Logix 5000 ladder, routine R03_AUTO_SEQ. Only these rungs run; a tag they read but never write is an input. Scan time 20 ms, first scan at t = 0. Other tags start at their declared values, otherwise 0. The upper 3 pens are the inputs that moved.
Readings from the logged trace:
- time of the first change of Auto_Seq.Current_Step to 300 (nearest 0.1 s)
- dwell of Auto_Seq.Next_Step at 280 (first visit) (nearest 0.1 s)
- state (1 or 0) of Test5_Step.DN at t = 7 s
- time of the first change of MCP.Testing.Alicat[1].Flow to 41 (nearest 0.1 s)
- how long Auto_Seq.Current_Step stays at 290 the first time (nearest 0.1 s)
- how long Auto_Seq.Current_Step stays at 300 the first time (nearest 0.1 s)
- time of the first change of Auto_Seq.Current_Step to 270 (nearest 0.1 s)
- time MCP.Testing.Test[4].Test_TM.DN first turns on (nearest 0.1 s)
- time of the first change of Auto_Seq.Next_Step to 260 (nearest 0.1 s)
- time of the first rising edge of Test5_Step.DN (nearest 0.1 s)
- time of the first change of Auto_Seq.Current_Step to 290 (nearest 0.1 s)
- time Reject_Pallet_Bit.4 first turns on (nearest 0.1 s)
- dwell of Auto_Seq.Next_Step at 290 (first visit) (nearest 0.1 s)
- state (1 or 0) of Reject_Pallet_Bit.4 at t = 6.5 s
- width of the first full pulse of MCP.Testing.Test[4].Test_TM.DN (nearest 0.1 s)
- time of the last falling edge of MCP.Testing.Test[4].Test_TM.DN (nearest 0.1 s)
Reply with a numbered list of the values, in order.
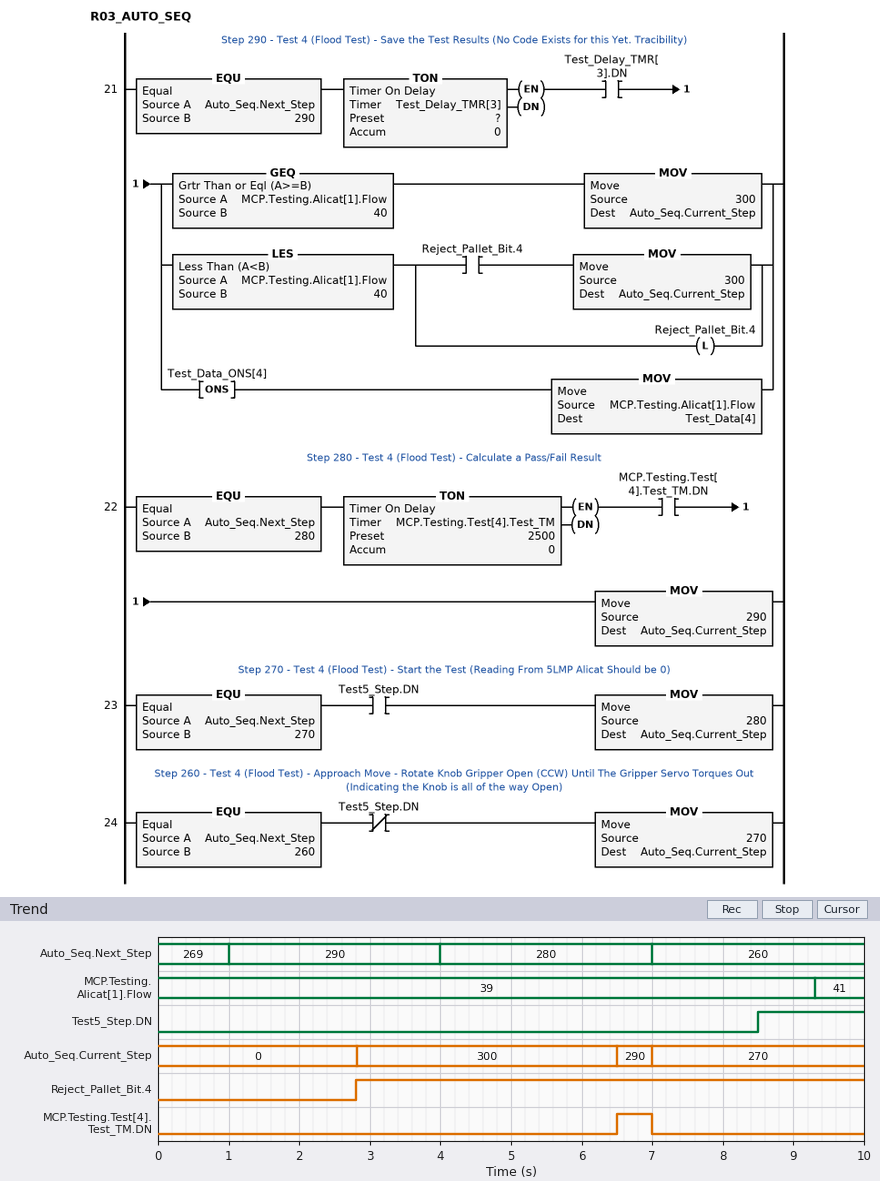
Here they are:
1. 2.8 s
2. 3.0 s
3. 0
4. 9.3 s
5. 0.5 s
6. 3.7 s
7. 7.0 s
8. 6.5 s
9. 7.0 s
10. 8.5 s
11. 6.5 s
12. 2.8 s
13. 3.0 s
14. 1
15. 0.5 s
16. 7.0 s
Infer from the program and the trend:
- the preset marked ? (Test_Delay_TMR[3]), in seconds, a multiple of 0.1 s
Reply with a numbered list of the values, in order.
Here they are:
1. 1.8 s
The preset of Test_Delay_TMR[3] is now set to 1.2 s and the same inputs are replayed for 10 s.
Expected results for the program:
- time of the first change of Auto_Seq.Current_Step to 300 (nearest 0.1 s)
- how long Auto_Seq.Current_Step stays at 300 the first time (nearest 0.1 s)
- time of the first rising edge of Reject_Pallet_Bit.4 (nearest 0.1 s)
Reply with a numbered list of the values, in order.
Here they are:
1. 2.2 s
2. 4.3 s
3. 2.2 s
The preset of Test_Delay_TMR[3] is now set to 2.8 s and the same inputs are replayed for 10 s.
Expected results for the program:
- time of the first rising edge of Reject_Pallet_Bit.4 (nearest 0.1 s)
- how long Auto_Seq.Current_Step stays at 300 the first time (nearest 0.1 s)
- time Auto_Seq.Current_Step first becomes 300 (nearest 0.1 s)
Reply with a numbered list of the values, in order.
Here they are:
1. 3.8 s
2. 2.7 s
3. 3.8 s
